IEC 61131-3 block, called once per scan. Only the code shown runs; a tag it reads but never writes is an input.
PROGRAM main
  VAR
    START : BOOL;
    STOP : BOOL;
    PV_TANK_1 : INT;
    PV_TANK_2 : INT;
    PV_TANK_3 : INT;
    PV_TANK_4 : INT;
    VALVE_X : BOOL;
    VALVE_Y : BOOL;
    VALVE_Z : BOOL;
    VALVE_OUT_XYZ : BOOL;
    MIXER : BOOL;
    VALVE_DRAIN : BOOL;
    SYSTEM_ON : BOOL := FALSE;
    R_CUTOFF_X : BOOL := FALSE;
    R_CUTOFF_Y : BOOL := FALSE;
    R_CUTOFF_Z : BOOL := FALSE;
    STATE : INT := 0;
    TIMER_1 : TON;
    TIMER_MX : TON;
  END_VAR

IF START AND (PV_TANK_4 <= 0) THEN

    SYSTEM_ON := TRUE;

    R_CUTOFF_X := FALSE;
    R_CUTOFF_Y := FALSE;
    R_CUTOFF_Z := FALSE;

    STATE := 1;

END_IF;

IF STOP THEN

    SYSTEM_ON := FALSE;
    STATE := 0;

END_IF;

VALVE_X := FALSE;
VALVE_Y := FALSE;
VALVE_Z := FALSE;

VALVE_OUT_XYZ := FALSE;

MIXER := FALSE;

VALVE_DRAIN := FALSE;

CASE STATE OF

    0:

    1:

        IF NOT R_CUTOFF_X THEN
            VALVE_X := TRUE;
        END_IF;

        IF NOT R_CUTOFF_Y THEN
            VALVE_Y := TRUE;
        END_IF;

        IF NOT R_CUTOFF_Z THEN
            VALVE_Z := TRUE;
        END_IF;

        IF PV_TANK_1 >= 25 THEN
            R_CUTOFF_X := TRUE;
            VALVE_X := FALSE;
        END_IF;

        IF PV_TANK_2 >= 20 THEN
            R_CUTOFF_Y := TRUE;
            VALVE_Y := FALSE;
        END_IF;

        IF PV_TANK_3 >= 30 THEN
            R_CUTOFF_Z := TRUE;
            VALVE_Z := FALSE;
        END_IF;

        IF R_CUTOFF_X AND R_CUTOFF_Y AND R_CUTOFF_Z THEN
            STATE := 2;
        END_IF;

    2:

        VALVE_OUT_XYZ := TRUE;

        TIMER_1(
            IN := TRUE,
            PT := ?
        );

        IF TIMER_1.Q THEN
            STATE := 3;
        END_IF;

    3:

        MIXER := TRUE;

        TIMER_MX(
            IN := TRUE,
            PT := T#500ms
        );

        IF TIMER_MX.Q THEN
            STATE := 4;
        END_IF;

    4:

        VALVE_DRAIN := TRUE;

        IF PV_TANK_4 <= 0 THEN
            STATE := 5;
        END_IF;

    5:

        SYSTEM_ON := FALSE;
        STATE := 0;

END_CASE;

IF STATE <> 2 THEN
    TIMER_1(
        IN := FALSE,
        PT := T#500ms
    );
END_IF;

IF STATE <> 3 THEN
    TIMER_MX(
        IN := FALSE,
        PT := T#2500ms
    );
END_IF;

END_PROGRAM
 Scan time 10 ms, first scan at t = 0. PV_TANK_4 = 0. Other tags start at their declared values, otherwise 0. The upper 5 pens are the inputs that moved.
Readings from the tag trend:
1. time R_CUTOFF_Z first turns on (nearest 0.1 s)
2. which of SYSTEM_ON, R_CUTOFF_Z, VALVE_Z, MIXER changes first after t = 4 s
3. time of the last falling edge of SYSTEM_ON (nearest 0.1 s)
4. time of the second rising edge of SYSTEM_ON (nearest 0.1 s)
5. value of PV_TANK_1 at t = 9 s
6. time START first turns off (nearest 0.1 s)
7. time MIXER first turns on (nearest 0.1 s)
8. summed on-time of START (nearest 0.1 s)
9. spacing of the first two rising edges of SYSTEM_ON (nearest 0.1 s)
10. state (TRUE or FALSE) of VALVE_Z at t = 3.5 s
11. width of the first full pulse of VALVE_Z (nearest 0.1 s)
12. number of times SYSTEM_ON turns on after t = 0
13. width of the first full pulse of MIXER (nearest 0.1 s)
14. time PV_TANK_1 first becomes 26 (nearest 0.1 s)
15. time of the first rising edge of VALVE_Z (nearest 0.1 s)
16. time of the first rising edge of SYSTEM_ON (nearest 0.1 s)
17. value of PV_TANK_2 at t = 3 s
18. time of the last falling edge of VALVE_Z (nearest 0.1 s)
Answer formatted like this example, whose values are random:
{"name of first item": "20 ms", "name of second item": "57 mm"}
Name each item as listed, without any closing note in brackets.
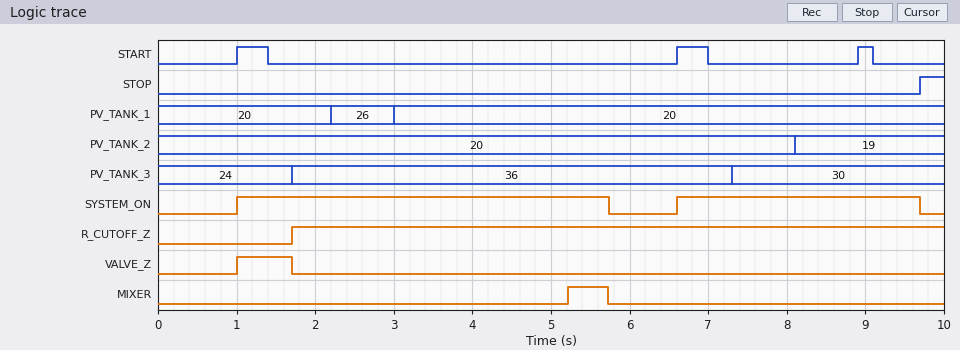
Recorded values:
{"time R_CUTOFF_Z first turns on": "1.7 s", "which of SYSTEM_ON, R_CUTOFF_Z, VALVE_Z, MIXER changes first after t = 4 s": "MIXER", "time of the last falling edge of SYSTEM_ON": "9.7 s", "time of the second rising edge of SYSTEM_ON": "6.6 s", "value of PV_TANK_1 at t = 9 s": "20", "time START first turns off": "1.4 s", "time MIXER first turns on": "5.2 s", "summed on-time of START": "1.0 s", "spacing of the first two rising edges of SYSTEM_ON": "5.6 s", "state (TRUE or FALSE) of VALVE_Z at t = 3.5 s": "FALSE", "width of the first full pulse of VALVE_Z": "0.7 s", "number of times SYSTEM_ON turns on after t = 0": "2", "width of the first full pulse of MIXER": "0.5 s", "time PV_TANK_1 first becomes 26": "2.2 s", "time of the first rising edge of VALVE_Z": "1.0 s", "time of the first rising edge of SYSTEM_ON": "1.0 s", "value of PV_TANK_2 at t = 3 s": "20", "time of the last falling edge of VALVE_Z": "1.7 s"}
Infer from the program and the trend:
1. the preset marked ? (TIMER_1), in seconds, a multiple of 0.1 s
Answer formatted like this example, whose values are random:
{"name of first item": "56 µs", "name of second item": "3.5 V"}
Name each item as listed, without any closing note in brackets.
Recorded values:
{"the preset marked ? (TIMER_1), in seconds, a multiple of 0.1 s": "3.0 s"}
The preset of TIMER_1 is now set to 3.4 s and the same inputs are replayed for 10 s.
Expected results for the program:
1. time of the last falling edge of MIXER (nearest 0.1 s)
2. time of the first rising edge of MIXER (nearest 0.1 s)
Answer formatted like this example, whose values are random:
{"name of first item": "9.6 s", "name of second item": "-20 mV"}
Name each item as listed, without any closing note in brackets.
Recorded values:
{"time of the last falling edge of MIXER": "6.1 s", "time of the first rising edge of MIXER": "5.6 s"}
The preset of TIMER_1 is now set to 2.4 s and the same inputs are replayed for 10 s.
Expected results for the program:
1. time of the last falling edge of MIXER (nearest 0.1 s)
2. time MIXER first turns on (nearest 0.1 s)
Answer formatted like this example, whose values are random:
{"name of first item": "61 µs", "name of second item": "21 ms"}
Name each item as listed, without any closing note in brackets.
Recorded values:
{"time of the last falling edge of MIXER": "5.1 s", "time MIXER first turns on": "4.6 s"}
